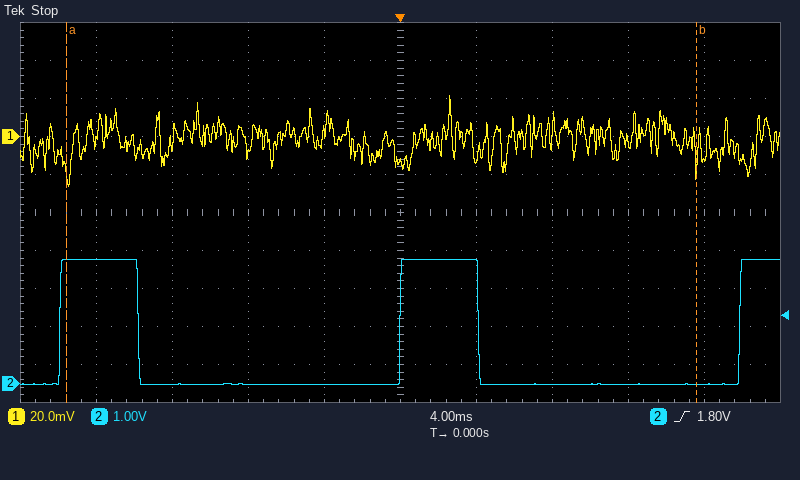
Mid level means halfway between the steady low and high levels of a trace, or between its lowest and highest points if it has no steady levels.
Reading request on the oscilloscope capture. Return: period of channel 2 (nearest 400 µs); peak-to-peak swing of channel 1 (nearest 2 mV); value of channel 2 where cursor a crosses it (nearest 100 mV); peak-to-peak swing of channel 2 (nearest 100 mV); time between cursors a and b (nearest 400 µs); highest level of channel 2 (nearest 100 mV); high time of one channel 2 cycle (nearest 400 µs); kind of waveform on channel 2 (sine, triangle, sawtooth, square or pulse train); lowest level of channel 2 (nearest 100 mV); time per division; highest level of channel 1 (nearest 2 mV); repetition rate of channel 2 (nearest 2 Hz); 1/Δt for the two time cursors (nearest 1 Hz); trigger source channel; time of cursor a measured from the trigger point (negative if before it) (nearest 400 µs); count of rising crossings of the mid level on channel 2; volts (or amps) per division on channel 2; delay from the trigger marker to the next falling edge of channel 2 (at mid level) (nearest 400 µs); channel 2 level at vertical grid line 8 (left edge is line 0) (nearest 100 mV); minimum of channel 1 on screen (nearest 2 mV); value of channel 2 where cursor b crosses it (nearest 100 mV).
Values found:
18.0 ms
48 mV
3.3 V
3.3 V
33.2 ms
3.3 V
4.0 ms
pulse train
0.0 V
4 ms
22 mV
56 Hz
30 Hz
channel 2
-17.6 ms
3
1 V
4.0 ms
0.0 V
-26 mV
0.0 V
